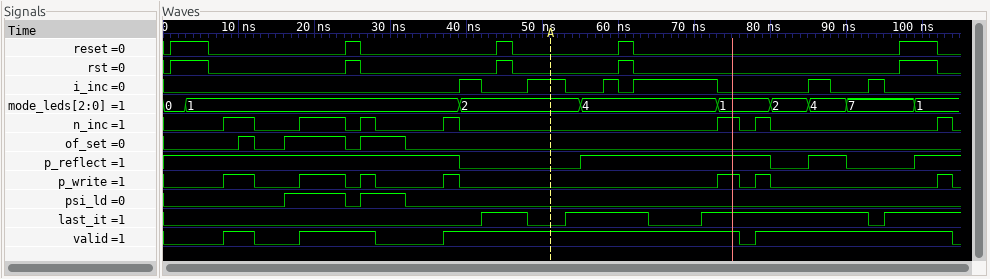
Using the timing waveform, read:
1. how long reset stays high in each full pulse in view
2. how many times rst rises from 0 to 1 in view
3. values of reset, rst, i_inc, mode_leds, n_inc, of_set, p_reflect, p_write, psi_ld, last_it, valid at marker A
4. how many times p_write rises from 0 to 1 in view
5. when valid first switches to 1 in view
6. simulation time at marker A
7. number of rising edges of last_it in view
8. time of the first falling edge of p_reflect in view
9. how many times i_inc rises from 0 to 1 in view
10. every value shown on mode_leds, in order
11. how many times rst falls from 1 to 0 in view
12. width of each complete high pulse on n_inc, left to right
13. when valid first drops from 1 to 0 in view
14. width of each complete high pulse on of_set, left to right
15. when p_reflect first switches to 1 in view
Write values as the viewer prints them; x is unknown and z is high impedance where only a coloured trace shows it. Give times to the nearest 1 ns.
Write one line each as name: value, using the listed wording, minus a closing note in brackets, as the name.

how long reset stays high in each full pulse in view: 5 ns, 2 ns, 2 ns, 2 ns, 5 ns
how many times rst rises from 0 to 1 in view: 5
values of reset, rst, i_inc, mode_leds, n_inc, of_set, p_reflect, p_write, psi_ld, last_it, valid at marker A: reset=0, rst=0, i_inc=1, mode_leds=2, n_inc=0, of_set=0, p_reflect=0, p_write=0, psi_ld=0, last_it=0, valid=1
how many times p_write rises from 0 to 1 in view: 7
when valid first switches to 1 in view: 8 ns
simulation time at marker A: 51 ns
number of rising edges of last_it in view: 4
time of the first falling edge of p_reflect in view: 39 ns
how many times i_inc rises from 0 to 1 in view: 6
every value shown on mode_leds, in order: 0, 1, 2, 4, 1, 2, 4, 7, 1
how many times rst falls from 1 to 0 in view: 5
width of each complete high pulse on n_inc, left to right: 4 ns, 6 ns, 2 ns, 2 ns, 3 ns, 2 ns, 2 ns
when valid first drops from 1 to 0 in view: 12 ns
width of each complete high pulse on of_set, left to right: 2 ns, 8 ns, 6 ns
when p_reflect first switches to 1 in view: 55 ns
